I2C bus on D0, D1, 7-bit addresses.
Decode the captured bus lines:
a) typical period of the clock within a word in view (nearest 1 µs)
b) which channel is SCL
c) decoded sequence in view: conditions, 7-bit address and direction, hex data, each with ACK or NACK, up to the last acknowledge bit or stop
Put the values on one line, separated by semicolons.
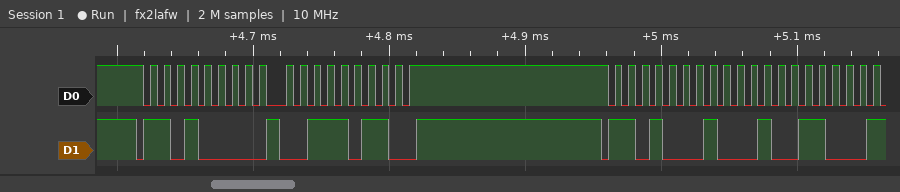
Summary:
10 µs; D0; start, address 68 write ACK, 3B ACK, stop, start, address 68 read ACK, 26 ACK
